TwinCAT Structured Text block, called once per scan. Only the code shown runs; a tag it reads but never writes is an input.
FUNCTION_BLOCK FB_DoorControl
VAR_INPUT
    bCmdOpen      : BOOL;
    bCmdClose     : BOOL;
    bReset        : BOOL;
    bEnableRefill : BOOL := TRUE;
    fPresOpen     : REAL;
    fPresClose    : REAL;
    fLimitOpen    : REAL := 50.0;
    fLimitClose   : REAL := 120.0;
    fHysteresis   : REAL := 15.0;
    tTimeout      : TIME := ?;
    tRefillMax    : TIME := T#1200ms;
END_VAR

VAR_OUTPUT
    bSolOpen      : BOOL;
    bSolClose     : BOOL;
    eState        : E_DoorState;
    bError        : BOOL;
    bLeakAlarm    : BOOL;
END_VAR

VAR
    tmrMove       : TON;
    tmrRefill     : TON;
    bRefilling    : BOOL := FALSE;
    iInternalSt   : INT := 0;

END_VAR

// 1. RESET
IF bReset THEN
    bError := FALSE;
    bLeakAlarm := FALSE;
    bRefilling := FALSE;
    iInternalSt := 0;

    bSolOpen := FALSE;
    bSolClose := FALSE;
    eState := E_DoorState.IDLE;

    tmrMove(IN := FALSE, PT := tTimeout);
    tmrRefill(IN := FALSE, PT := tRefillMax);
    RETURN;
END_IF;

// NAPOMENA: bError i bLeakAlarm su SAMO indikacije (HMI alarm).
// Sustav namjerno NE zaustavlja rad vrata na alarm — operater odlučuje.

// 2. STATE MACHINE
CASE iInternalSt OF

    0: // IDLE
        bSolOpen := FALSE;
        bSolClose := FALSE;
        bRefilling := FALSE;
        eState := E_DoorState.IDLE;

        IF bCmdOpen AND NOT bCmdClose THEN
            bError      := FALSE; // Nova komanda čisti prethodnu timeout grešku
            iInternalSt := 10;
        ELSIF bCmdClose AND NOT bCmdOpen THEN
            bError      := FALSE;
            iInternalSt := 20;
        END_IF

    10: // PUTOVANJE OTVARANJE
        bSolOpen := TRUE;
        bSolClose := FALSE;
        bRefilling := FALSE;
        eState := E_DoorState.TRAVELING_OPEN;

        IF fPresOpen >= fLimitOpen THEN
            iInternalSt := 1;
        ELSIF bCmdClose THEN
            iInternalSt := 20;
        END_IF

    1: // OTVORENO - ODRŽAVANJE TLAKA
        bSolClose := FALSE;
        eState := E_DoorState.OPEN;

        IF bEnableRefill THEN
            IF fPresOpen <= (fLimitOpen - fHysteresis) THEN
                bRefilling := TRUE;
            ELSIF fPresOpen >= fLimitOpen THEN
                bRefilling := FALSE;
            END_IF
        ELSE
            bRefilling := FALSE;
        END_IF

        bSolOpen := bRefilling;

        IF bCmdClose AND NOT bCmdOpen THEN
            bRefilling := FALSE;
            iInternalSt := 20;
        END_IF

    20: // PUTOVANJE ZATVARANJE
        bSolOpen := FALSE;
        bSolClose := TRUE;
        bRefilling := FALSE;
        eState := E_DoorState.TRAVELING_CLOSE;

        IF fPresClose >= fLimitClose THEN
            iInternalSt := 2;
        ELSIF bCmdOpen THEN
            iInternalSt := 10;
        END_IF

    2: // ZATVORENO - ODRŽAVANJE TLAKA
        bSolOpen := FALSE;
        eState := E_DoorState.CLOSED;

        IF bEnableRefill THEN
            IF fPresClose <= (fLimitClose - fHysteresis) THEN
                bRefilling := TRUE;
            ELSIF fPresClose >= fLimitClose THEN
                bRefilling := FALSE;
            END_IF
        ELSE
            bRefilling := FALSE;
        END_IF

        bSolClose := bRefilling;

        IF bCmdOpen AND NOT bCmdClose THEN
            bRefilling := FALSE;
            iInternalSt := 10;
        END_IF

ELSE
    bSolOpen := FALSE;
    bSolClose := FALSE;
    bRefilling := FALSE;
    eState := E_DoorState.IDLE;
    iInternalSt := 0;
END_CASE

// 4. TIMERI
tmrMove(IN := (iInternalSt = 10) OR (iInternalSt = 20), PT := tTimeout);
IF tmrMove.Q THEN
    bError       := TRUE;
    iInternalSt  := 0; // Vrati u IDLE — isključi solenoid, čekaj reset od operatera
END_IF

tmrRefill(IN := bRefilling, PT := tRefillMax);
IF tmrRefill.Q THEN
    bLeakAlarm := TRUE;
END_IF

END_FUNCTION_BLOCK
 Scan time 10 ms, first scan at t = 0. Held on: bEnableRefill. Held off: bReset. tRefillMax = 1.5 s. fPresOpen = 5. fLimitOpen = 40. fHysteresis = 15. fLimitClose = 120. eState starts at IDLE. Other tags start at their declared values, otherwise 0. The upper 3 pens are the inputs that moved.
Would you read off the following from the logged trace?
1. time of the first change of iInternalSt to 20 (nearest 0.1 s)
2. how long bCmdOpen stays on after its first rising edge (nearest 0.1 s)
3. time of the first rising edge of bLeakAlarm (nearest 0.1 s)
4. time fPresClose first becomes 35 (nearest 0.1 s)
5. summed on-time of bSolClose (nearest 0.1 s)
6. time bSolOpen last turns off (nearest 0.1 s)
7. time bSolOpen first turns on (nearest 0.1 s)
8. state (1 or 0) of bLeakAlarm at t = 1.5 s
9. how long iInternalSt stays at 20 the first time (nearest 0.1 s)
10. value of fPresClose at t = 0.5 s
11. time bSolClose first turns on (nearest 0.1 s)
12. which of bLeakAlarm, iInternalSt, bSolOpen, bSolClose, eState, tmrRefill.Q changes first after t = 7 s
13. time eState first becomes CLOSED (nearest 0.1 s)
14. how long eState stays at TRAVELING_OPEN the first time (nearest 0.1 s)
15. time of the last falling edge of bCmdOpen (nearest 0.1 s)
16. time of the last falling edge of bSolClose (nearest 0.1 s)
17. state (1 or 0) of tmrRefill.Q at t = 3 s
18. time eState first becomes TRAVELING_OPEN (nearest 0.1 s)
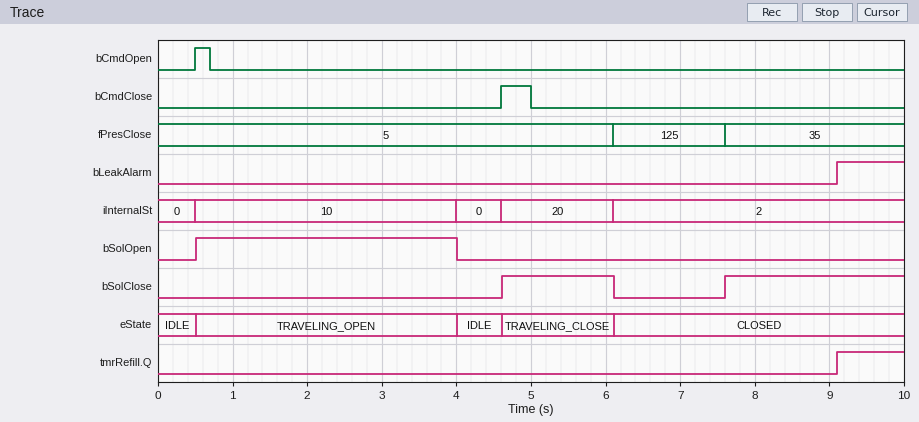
4.6 s
0.2 s
9.1 s
7.6 s
3.9 s
4.0 s
0.5 s
0
1.5 s
5
4.6 s
bSolClose
6.1 s
3.5 s
0.7 s
6.1 s
0
0.5 s
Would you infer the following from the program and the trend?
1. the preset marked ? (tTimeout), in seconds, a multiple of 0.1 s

3.5 s
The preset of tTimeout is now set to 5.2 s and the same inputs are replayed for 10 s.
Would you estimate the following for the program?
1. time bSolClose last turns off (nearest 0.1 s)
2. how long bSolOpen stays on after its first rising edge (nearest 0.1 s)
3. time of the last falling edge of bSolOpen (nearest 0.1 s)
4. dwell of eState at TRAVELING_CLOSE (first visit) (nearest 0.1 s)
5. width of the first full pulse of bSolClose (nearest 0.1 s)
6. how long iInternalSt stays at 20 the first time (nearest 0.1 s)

5.7 s
4.1 s
4.6 s
1.1 s
1.1 s
1.1 s
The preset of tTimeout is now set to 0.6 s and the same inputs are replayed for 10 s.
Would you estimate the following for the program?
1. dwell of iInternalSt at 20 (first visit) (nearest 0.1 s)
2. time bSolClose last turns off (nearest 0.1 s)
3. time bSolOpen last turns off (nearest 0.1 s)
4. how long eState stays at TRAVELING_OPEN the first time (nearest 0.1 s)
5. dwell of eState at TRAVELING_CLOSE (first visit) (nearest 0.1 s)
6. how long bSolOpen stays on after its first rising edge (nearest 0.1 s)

0.6 s
5.2 s
1.1 s
0.6 s
0.6 s
0.6 s
